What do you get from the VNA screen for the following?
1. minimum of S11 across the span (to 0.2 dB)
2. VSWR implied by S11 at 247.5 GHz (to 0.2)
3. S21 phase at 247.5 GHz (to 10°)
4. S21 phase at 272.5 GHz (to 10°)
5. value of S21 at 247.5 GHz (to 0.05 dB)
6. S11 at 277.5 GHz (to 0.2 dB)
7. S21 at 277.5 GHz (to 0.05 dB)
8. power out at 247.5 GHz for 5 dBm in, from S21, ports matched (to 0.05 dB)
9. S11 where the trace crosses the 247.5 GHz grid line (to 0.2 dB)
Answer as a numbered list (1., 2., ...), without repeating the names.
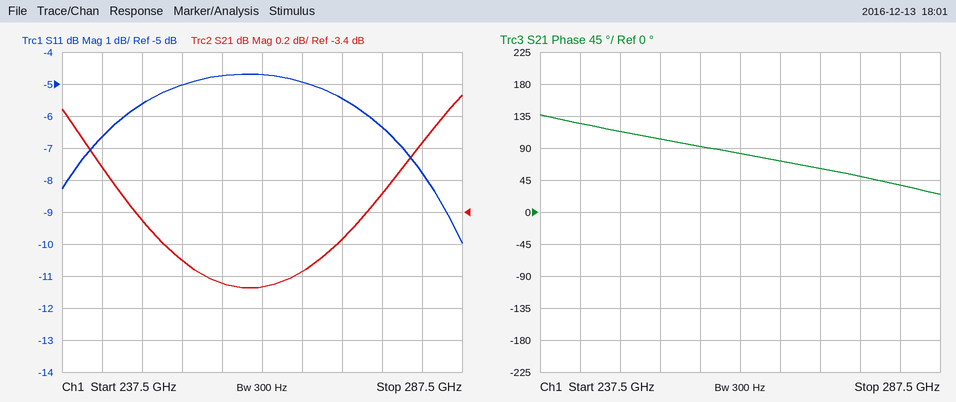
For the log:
1. -10.0 dB
2. 3.2
3. 110°
4. 60°
5. -3.45 dB
6. -6.4 dB
7. -3.30 dB
8. 1.55 dBm
9. -5.6 dB
